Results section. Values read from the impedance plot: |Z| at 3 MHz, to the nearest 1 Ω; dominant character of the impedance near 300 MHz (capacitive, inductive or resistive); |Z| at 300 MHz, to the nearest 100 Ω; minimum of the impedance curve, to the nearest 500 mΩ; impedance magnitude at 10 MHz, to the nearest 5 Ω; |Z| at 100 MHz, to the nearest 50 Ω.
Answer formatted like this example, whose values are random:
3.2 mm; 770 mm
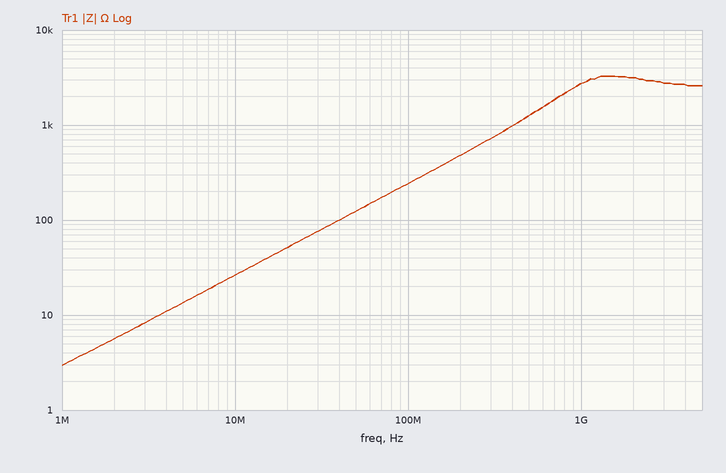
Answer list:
8 Ω; inductive; 700 Ω; 3.0 Ω; 25 Ω; 250 Ω
